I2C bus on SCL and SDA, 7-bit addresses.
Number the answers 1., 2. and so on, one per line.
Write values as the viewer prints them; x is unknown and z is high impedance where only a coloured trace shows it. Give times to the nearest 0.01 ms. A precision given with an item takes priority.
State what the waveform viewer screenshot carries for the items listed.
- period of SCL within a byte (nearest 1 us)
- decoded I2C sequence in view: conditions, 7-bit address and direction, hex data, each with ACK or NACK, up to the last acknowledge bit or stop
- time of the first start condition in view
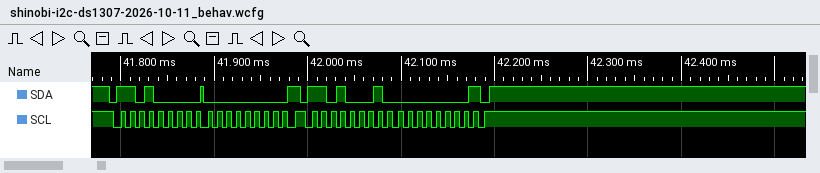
1. 10 us
2. start, address 68 write ACK, 00 ACK, repeated start, address 68 read ACK, 00 NACK, stop
3. 41.79 ms
